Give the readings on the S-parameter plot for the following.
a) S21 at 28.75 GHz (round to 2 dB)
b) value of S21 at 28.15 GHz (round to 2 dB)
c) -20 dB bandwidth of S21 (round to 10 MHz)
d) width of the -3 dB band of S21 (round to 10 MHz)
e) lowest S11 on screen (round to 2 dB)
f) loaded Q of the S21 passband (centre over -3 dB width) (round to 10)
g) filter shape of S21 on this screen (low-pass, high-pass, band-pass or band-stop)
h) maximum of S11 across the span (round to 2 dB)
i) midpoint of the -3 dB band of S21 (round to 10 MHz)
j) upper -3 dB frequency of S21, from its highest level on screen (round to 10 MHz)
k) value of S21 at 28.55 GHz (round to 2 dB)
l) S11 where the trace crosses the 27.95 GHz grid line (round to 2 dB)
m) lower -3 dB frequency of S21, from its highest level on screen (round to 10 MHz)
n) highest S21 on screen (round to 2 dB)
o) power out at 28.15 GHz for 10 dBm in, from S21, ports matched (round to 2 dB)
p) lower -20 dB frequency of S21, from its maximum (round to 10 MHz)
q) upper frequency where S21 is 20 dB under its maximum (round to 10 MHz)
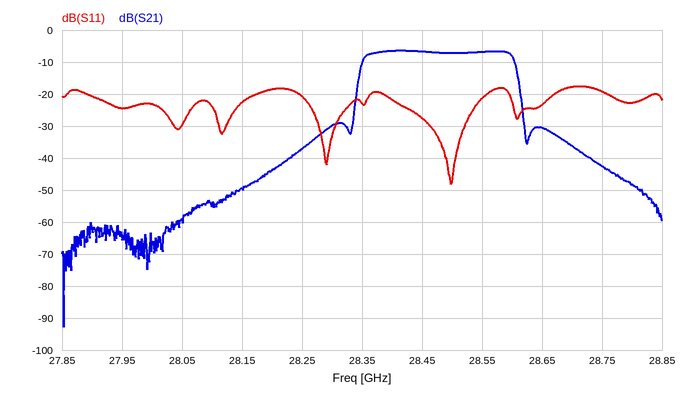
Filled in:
-42 dB
-50 dB
280 MHz
250 MHz
-48 dB
110
band-pass
-18 dB
28.48 GHz
28.60 GHz
-6 dB
-24 dB
28.35 GHz
-6 dB
-40 dBm
28.34 GHz
28.62 GHz
